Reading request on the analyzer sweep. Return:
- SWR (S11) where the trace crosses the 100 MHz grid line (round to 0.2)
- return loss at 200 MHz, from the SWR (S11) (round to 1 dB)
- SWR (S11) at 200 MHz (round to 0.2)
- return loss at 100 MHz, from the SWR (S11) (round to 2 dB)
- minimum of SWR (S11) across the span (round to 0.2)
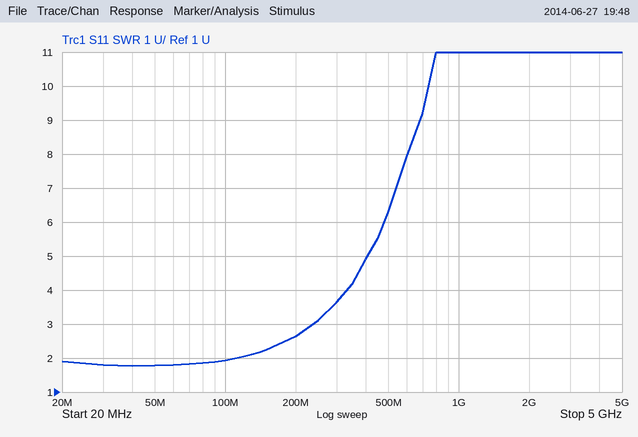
2.0
7 dB
2.6
10 dB
1.8
